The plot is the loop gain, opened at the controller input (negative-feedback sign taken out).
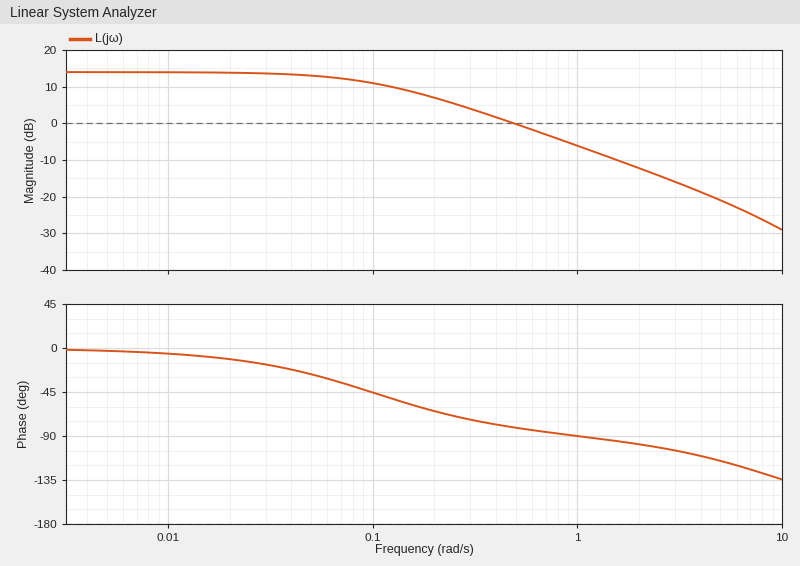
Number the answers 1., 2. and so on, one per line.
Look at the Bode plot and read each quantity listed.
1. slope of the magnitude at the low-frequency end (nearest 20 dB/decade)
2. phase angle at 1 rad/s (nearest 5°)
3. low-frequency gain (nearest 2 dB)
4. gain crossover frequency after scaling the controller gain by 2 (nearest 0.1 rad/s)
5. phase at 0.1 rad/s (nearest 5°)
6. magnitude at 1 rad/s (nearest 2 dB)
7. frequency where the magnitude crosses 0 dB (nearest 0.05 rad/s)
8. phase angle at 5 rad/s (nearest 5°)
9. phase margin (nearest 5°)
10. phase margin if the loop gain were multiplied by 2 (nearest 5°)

1. 0 dB/decade
2. -90°
3. 14 dB
4. 1.0 rad/s
5. -45°
6. -6 dB
7. 0.50 rad/s
8. -115°
9. 100°
10. 90°
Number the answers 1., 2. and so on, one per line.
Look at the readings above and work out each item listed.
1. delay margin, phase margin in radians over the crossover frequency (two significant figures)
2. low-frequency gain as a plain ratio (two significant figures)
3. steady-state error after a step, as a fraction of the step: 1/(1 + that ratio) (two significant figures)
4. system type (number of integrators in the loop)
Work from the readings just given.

1. 3.5 s
2. 5.0
3. 0.17
4. 0
